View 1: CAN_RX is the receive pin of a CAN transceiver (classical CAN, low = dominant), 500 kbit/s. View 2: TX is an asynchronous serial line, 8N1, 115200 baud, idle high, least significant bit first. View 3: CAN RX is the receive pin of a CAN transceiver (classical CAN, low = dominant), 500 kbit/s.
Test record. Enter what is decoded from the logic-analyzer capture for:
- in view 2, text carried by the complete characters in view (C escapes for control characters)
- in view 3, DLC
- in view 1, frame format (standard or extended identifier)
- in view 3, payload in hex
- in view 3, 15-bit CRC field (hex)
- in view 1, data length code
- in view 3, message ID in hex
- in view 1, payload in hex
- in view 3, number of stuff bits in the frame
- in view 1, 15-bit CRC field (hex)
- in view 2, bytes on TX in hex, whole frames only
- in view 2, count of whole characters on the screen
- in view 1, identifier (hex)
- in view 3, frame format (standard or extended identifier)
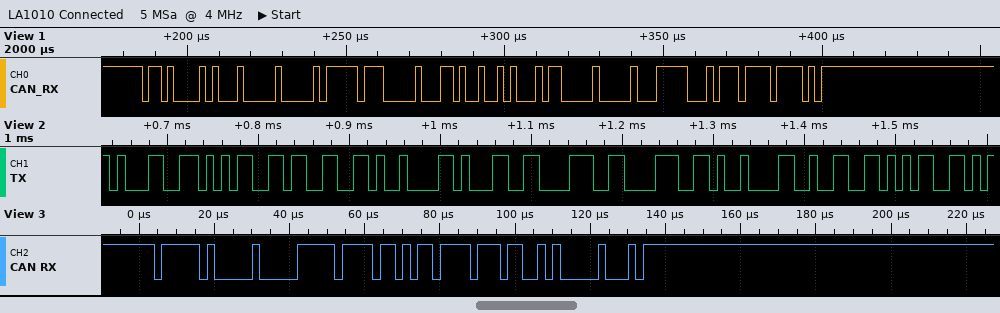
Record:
"153\t188\t25"
3
standard
FD AD EE
0x6500
8
0x7E0
00 FF 00 D2 51 60 00 F9
5
0x3BDE
31 35 33 09 31 38 38 09 32 35
10
0x685
standard
